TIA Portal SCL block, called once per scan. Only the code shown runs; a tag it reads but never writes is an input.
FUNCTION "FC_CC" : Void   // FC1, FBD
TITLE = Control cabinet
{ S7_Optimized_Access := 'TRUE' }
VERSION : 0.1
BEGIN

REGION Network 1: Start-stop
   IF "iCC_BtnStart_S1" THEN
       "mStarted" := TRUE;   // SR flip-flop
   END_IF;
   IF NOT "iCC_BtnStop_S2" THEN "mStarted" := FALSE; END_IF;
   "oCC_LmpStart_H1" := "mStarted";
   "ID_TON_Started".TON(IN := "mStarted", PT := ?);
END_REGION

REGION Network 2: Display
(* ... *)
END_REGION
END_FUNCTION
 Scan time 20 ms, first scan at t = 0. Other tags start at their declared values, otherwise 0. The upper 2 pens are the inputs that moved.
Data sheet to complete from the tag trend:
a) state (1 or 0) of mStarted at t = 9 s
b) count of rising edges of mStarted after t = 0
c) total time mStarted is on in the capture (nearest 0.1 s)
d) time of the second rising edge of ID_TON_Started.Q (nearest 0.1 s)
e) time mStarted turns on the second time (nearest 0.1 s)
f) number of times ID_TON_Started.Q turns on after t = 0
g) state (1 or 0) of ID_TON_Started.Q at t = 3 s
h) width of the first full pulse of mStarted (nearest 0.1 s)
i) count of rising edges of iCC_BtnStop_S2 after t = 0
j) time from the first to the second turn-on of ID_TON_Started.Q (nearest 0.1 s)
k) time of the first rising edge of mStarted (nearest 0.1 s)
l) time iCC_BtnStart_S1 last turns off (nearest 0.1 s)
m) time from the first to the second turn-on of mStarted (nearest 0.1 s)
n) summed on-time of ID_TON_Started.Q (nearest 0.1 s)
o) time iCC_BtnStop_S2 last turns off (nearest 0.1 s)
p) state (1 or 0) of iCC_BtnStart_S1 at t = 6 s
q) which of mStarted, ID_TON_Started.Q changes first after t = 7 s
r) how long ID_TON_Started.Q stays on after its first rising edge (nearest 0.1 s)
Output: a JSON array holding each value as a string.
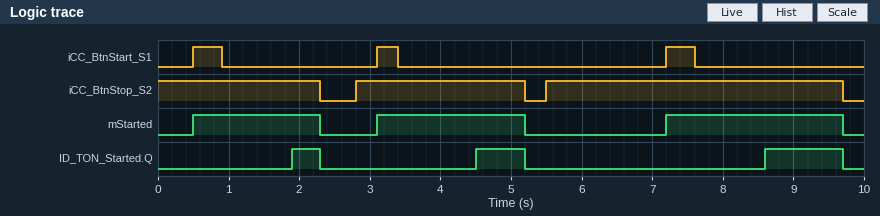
["1", "3", "6.4 s", "4.5 s", "3.1 s", "3", "0", "1.8 s", "2", "2.6 s", "0.5 s", "7.6 s", "2.6 s", "2.2 s", "9.7 s", "0", "mStarted", "0.4 s"]
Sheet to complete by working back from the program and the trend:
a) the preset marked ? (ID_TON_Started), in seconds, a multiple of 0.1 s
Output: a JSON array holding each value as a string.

["1.4 s"]
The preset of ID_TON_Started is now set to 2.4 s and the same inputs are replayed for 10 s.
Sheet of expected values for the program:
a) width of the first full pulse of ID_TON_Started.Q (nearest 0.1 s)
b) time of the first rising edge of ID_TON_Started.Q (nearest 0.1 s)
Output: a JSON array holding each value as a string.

["0.1 s", "9.6 s"]
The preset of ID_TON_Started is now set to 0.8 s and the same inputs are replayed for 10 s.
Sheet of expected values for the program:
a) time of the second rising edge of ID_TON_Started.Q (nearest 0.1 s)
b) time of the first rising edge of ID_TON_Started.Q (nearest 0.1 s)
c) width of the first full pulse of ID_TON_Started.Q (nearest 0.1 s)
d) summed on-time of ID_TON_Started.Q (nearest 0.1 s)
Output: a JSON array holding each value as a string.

["3.9 s", "1.3 s", "1.0 s", "4.0 s"]
